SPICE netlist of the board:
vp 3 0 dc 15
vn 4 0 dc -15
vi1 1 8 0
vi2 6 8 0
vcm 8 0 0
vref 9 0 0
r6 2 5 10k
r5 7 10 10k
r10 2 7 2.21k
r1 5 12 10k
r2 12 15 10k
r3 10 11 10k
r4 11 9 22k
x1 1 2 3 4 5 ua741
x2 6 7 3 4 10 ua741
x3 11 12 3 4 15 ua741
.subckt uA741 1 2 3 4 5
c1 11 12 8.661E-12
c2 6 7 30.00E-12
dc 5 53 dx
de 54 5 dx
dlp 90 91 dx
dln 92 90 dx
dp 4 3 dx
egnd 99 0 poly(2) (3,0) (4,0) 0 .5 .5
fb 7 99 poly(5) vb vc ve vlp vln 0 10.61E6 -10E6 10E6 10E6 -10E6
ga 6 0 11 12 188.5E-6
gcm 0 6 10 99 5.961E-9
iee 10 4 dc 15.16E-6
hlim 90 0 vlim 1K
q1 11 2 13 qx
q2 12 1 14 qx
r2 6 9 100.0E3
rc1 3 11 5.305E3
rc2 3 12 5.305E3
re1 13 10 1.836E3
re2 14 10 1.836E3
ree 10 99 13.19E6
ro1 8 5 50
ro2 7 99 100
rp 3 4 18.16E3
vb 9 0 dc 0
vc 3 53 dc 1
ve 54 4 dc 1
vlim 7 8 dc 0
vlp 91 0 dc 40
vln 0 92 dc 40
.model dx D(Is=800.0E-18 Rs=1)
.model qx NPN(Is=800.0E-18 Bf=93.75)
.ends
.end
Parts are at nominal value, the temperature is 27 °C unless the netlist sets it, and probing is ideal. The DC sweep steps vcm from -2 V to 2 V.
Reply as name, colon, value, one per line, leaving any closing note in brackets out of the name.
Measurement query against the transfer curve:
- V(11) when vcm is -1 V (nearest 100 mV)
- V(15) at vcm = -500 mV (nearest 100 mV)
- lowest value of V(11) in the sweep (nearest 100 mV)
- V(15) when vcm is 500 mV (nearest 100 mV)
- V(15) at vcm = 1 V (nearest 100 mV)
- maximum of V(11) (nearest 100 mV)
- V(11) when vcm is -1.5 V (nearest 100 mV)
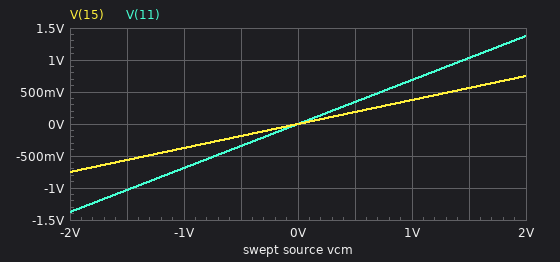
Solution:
V(11) when vcm is -1 V: -700 mV
V(15) at vcm = -500 mV: -200 mV
lowest value of V(11) in the sweep: -1.4 V
V(15) when vcm is 500 mV: 200 mV
V(15) at vcm = 1 V: 400 mV
maximum of V(11): 1.4 V
V(11) when vcm is -1.5 V: -1.0 V
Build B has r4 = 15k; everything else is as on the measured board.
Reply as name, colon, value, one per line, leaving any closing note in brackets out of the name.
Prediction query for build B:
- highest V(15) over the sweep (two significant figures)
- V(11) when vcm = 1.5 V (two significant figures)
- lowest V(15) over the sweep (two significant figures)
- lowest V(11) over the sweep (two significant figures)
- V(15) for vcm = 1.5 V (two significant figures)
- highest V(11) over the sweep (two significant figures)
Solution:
highest V(15) over the sweep: 400 mV
V(11) when vcm = 1.5 V: 900 mV
lowest V(15) over the sweep: -400 mV
lowest V(11) over the sweep: -1.2 V
V(15) for vcm = 1.5 V: 300 mV
highest V(11) over the sweep: 1.2 V
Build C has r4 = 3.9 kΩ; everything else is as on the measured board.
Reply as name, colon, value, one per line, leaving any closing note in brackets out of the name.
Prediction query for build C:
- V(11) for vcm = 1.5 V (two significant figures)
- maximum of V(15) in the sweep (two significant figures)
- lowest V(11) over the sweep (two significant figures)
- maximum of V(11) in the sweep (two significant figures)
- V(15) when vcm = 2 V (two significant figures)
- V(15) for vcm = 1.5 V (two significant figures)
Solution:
V(11) for vcm = 1.5 V: 420 mV
maximum of V(15) in the sweep: 880 mV
lowest V(11) over the sweep: -560 mV
maximum of V(11) in the sweep: 560 mV
V(15) when vcm = 2 V: -880 mV
V(15) for vcm = 1.5 V: -660 mV
